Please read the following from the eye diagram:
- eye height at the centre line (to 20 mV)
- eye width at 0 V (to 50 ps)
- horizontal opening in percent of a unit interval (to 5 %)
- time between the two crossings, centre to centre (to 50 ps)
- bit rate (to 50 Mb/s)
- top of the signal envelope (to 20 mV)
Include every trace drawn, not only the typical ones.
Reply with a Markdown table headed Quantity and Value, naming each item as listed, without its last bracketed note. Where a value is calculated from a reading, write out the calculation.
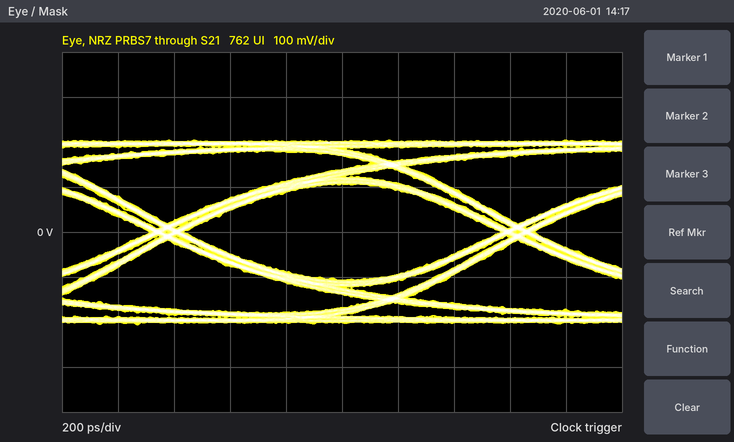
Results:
| Quantity | Value |
|---|---|
| eye height at the centre line | 220 mV |
| eye width at 0 V | 1.15 ns |
| horizontal opening in percent of a unit interval | 1.15 ns / 1.25 ns ≈ 92.0 %, so 90 % to the nearest 5 % |
| time between the two crossings, centre to centre | 1.25 ns |
| bit rate | 800 Mb/s |
| top of the signal envelope | 200 mV |
